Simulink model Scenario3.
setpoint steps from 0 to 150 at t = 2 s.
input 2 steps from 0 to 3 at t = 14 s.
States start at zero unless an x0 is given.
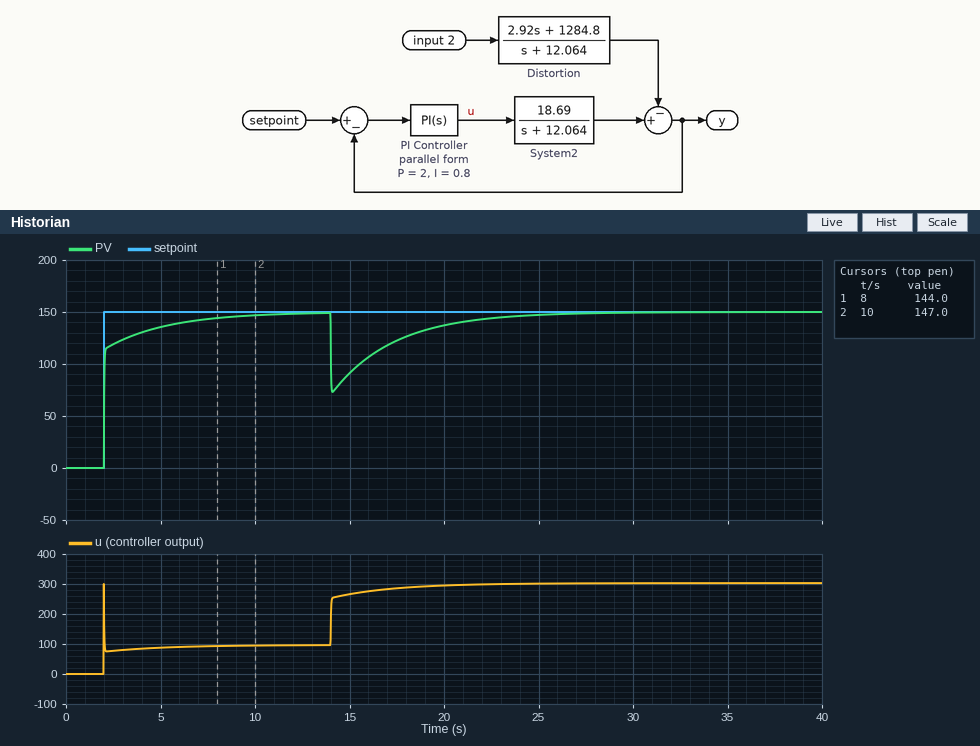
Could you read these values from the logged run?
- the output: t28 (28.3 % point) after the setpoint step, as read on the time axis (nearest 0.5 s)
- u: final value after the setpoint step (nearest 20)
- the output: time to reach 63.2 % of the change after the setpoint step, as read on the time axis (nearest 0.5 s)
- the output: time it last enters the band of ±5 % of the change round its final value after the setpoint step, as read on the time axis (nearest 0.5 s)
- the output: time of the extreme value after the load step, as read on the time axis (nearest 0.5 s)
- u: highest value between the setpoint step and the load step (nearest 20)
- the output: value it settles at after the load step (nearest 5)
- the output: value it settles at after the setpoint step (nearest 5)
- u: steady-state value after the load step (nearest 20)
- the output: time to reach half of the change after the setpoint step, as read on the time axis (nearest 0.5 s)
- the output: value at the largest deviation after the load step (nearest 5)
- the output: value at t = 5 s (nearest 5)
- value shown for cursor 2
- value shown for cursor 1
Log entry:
2.0 s
100
2.0 s
7.0 s
14.0 s
300
150
150
300
2.0 s
75
135
147.0
144.0
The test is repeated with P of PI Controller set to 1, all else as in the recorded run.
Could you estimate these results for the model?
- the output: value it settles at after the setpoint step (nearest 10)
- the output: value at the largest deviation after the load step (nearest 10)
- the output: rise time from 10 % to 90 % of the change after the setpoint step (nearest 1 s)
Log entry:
150
30
3 s
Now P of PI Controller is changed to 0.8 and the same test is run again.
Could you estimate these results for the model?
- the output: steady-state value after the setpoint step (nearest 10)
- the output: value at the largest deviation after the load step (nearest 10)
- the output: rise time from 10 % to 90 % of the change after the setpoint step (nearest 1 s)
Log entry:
150
20
3 s
